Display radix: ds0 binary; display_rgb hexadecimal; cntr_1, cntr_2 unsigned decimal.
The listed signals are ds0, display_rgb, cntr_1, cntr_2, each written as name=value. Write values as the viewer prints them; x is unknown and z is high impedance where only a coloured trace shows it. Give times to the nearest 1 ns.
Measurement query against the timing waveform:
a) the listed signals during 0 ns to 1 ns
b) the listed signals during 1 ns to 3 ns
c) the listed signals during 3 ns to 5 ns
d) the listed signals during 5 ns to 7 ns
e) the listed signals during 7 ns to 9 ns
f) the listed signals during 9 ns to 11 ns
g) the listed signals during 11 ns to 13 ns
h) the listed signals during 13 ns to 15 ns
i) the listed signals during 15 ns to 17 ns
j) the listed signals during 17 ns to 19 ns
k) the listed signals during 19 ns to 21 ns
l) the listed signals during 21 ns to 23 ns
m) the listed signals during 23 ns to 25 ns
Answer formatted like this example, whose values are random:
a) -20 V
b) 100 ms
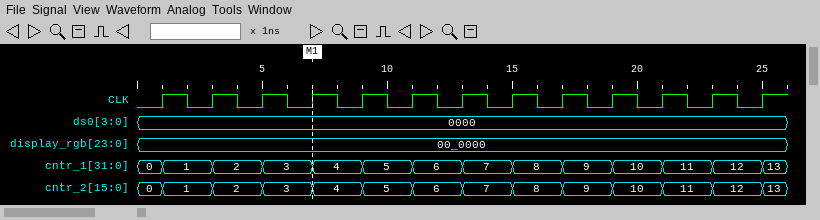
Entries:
a) ds0=0000, display_rgb=00_0000, cntr_1=0, cntr_2=0
b) ds0=0000, display_rgb=00_0000, cntr_1=1, cntr_2=1
c) ds0=0000, display_rgb=00_0000, cntr_1=2, cntr_2=2
d) ds0=0000, display_rgb=00_0000, cntr_1=3, cntr_2=3
e) ds0=0000, display_rgb=00_0000, cntr_1=4, cntr_2=4
f) ds0=0000, display_rgb=00_0000, cntr_1=5, cntr_2=5
g) ds0=0000, display_rgb=00_0000, cntr_1=6, cntr_2=6
h) ds0=0000, display_rgb=00_0000, cntr_1=7, cntr_2=7
i) ds0=0000, display_rgb=00_0000, cntr_1=8, cntr_2=8
j) ds0=0000, display_rgb=00_0000, cntr_1=9, cntr_2=9
k) ds0=0000, display_rgb=00_0000, cntr_1=10, cntr_2=10
l) ds0=0000, display_rgb=00_0000, cntr_1=11, cntr_2=11
m) ds0=0000, display_rgb=00_0000, cntr_1=12, cntr_2=12
